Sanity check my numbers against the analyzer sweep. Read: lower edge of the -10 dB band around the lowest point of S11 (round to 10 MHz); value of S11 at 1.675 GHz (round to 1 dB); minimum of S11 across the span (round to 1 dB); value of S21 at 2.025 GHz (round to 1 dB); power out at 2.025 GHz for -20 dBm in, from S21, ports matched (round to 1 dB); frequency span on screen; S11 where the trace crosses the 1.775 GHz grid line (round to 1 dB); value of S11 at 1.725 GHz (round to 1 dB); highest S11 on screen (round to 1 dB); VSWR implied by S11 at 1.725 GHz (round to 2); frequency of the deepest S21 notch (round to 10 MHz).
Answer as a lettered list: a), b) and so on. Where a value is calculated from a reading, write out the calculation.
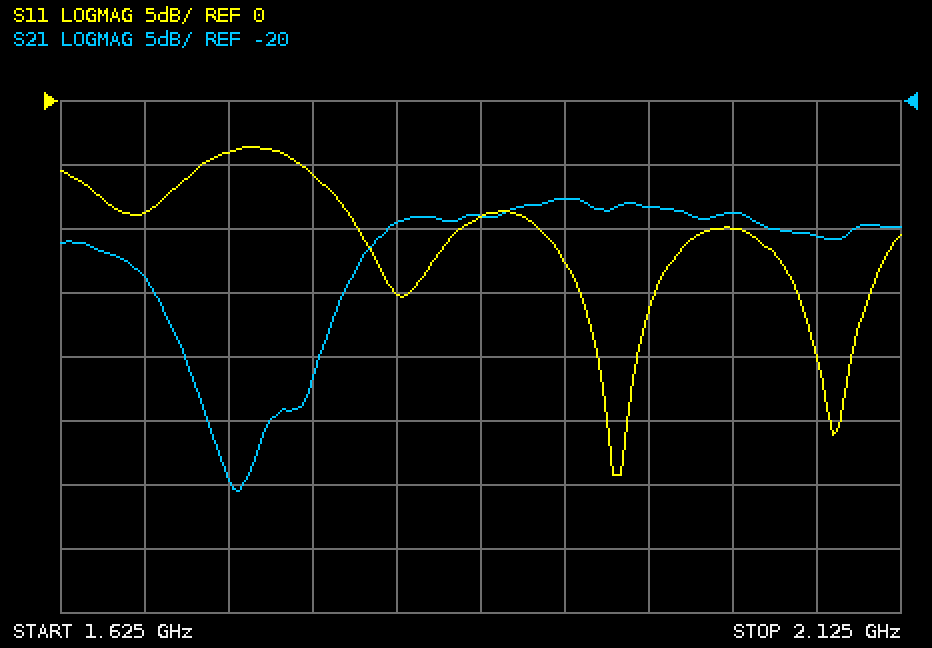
a) 1.91 GHz
b) -9 dB
c) -29 dB
d) -29 dB
e) -20 dBm + (-29 dB) = -49 dBm
f) 500 MHz
g) -6 dB
h) -4 dB
i) -4 dB
j) |Γ| = 10^(-4/20) = 0.6310; VSWR = (1 + 0.6310)/(1 − 0.6310) ≈ 4
k) 1.73 GHz
